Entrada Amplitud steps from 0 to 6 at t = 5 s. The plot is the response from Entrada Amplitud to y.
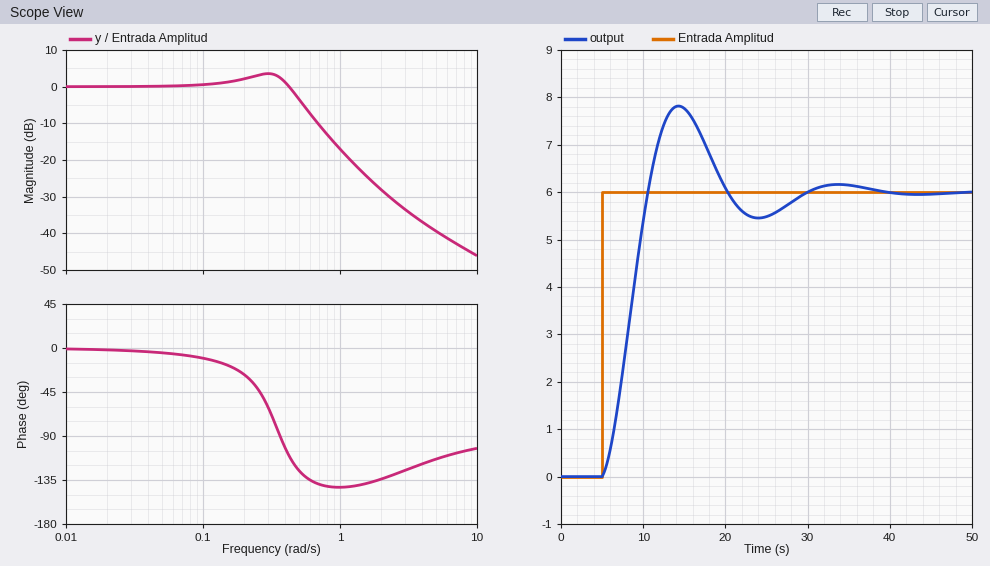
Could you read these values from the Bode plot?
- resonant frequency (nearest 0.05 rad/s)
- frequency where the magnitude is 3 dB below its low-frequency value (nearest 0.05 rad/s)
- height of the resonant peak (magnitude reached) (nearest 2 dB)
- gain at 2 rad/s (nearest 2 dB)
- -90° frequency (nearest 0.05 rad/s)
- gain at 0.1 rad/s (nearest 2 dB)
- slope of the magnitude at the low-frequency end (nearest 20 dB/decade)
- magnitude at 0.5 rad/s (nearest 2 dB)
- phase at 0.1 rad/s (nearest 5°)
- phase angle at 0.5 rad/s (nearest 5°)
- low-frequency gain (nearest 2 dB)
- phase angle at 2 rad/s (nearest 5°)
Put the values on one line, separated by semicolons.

0.30 rad/s; 0.50 rad/s; 4 dB; -28 dB; 0.35 rad/s; 0 dB; 0 dB/decade; -4 dB; -10°; -125°; 0 dB; -135°
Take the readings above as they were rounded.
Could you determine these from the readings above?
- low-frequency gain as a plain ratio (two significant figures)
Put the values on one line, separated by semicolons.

1.0
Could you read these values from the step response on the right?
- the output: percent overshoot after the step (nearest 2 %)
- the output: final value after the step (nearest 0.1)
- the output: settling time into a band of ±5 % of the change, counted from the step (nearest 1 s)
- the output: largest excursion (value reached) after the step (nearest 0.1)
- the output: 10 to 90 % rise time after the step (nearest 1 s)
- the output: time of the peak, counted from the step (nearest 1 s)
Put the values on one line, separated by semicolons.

30 %; 6.0; 22 s; 7.8; 4 s; 9 s
